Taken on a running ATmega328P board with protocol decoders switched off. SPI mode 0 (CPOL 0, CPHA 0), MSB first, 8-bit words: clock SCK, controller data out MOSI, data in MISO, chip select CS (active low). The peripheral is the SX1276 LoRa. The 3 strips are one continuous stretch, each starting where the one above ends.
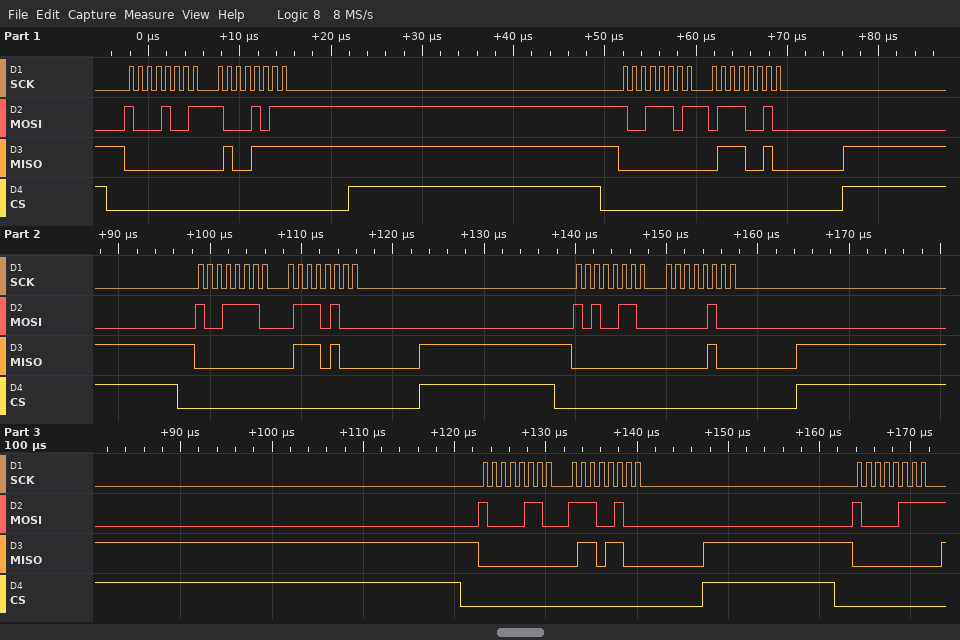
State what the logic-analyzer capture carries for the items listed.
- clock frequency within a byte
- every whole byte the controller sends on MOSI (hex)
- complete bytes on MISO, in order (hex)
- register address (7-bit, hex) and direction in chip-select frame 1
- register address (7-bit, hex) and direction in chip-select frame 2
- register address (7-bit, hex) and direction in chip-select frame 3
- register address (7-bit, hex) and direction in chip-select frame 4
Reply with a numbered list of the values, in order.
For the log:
1. 1 MHz
2. 89 8B 9D 72 9E 74 A6 04 86 E4 87
3. 00 4F 00 72 00 74 00 04 00 6C 00
4. 0x09 write
5. 0x1D write
6. 0x1E write
7. 0x26 write
